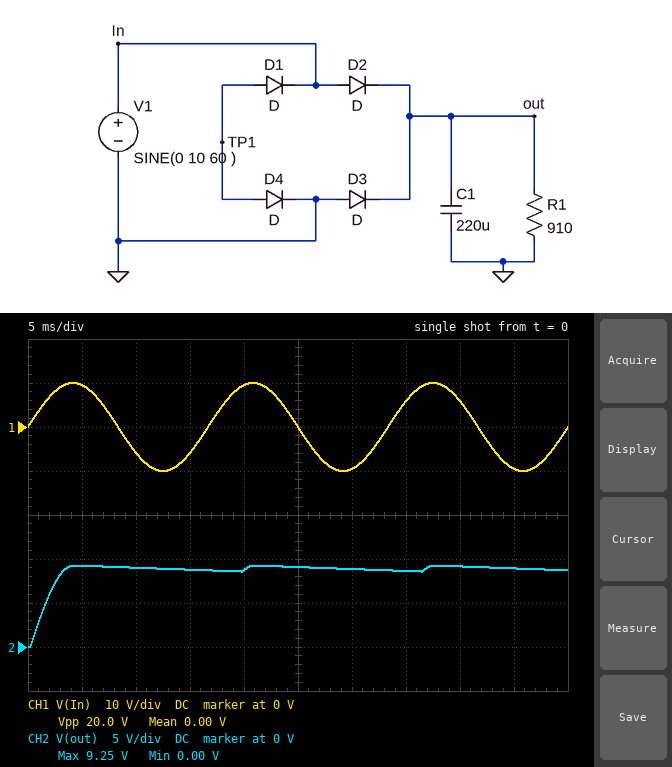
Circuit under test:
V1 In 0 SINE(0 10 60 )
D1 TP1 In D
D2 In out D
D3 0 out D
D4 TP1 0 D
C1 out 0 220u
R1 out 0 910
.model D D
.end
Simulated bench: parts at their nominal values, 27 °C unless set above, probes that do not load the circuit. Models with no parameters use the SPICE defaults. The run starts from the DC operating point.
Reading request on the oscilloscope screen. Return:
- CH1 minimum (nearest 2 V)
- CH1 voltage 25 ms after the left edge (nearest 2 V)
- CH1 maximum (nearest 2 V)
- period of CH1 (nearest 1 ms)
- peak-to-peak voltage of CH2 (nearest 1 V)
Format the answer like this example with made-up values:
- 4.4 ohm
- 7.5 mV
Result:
- -10 V
- 0 V
- 10 V
- 17 ms
- 9 V
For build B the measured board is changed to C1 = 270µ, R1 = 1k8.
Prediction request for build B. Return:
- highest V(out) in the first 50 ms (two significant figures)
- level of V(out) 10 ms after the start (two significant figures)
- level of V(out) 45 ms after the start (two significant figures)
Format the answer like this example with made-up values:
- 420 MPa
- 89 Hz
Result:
- 9.3 V
- 9.2 V
- 9.1 V
